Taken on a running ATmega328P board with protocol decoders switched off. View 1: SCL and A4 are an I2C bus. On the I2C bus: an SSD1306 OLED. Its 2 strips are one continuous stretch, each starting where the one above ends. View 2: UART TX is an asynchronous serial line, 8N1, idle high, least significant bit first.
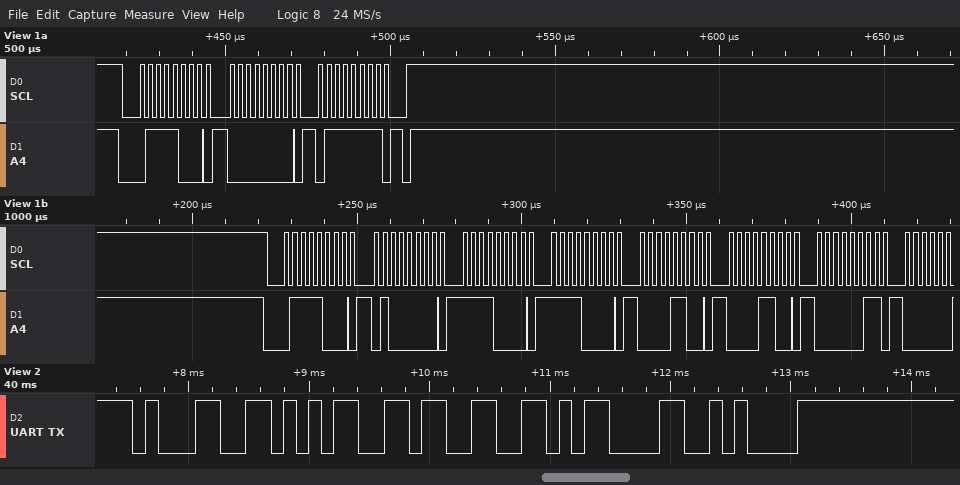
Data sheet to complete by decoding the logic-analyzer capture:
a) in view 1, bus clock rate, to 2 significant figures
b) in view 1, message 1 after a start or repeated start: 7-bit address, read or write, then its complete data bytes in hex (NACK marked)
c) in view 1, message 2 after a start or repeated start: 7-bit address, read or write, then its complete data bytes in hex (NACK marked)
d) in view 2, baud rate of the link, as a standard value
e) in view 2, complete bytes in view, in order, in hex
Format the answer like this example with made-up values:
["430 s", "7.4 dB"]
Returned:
["400 kHz", "0x3C write: 00 7F", "0x3C write: 40 F0 F0 0C 0C 03", "9600 baud", "0x31 0x35 0x33 0x0D 0x0A"]
